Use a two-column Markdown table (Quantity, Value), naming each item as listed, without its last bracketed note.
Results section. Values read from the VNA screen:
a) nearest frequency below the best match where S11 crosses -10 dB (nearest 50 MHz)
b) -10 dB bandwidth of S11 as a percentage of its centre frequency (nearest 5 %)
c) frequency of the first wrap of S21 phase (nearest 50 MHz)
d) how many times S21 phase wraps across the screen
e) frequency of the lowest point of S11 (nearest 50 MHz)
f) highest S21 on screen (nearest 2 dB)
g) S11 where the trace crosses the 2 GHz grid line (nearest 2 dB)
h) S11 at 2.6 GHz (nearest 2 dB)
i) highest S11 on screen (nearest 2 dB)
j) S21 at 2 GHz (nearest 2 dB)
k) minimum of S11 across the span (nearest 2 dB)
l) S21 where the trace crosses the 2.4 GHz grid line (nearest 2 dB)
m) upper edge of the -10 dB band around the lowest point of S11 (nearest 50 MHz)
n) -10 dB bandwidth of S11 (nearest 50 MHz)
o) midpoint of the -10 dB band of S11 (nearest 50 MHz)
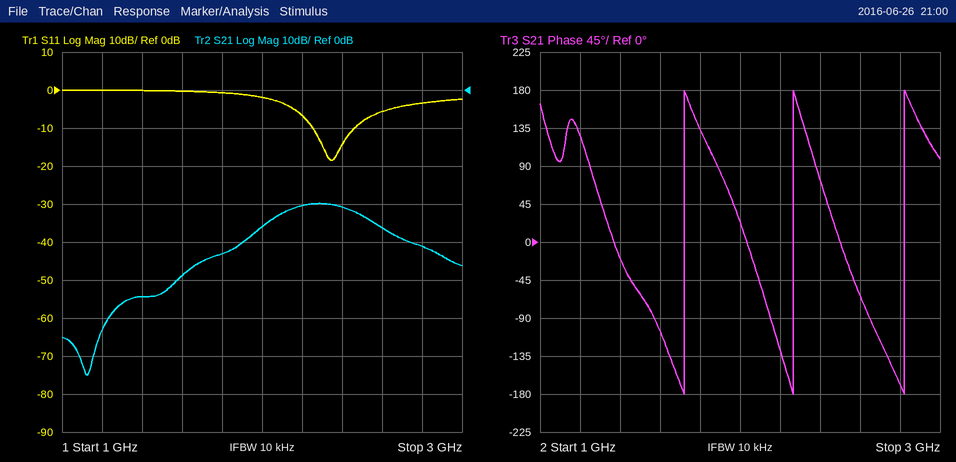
| Quantity | Value |
|---|---|
| nearest frequency below the best match where S11 crosses -10 dB | 2.25 GHz |
| -10 dB bandwidth of S11 as a percentage of its centre frequency | 10 % |
| frequency of the first wrap of S21 phase | 1.70 GHz |
| how many times S21 phase wraps across the screen | 3 |
| frequency of the lowest point of S11 | 2.35 GHz |
| highest S21 on screen | -30 dB |
| S11 where the trace crosses the 2 GHz grid line | -2 dB |
| S11 at 2.6 GHz | -6 dB |
| highest S11 on screen | 0 dB |
| S21 at 2 GHz | -36 dB |
| minimum of S11 across the span | -18 dB |
| S21 where the trace crosses the 2.4 GHz grid line | -30 dB |
| upper edge of the -10 dB band around the lowest point of S11 | 2.45 GHz |
| -10 dB bandwidth of S11 | 200 MHz |
| midpoint of the -10 dB band of S11 | 2.35 GHz |
